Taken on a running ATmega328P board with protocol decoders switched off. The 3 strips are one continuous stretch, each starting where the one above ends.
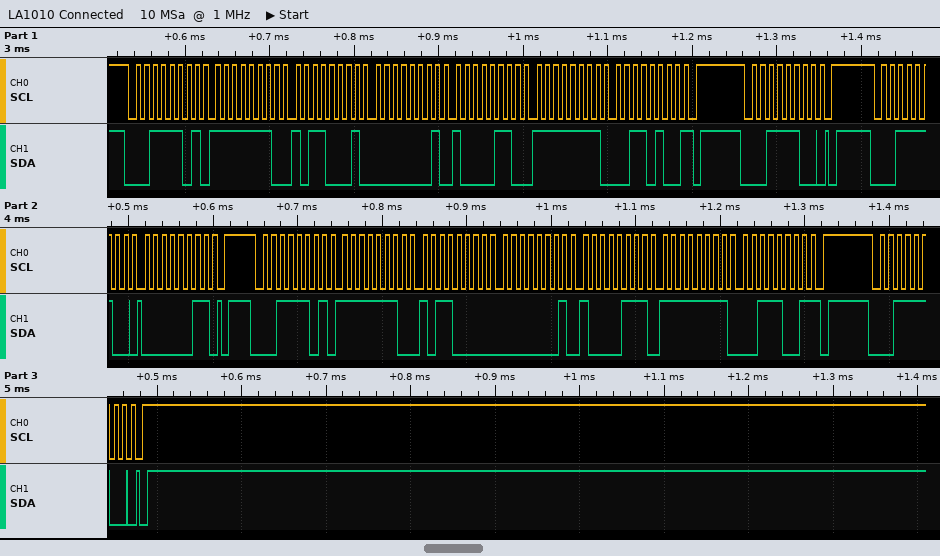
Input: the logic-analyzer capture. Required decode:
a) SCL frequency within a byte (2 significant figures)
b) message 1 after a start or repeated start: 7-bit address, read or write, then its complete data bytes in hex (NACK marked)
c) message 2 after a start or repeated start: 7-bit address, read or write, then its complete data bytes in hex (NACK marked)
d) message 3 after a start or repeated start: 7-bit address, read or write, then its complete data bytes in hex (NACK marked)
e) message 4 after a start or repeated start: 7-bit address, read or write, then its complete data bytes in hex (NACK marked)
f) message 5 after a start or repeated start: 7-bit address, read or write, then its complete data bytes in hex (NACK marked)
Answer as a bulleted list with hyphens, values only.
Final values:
- 100 kHz
- 0x1E read: FE B1 01 86 FF 34 NACK
- 0x1E write
- 0x1E write: 03
- 0x1E read: FE B0 01 87 FF 39 NACK
- 0x1E write
